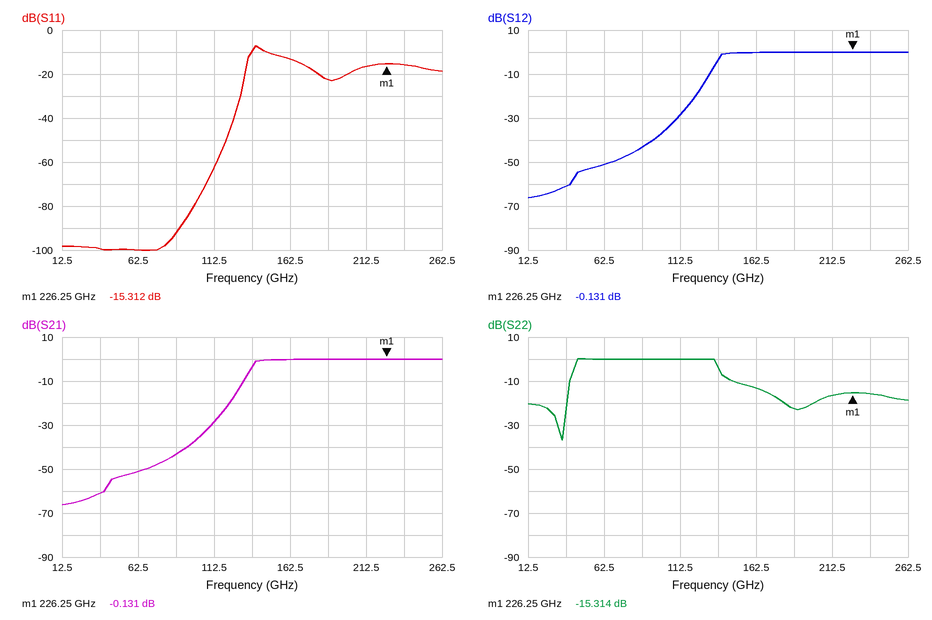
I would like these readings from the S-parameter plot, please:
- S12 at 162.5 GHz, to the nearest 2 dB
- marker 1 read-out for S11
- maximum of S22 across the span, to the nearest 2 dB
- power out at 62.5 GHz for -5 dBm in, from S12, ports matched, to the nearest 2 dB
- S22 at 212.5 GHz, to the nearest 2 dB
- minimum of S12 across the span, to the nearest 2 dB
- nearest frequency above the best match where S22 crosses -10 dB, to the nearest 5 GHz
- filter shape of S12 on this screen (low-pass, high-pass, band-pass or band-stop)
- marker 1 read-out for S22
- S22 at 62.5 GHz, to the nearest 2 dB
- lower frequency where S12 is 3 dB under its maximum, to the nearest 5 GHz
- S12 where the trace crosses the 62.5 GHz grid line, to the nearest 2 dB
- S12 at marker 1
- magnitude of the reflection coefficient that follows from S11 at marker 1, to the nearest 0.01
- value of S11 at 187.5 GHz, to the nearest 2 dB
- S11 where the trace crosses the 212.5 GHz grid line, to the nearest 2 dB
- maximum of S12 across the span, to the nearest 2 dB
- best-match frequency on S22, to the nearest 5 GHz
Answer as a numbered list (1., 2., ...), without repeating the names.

1. 0 dB
2. -15.312 dB
3. 0 dB
4. -56 dBm
5. -16 dB
6. -66 dB
7. 40 GHz
8. high-pass
9. -15.314 dB
10. 0 dB
11. 140 GHz
12. -52 dB
13. -0.131 dB
14. 0.17
15. -22 dB
16. -16 dB
17. 0 dB
18. 35 GHz
